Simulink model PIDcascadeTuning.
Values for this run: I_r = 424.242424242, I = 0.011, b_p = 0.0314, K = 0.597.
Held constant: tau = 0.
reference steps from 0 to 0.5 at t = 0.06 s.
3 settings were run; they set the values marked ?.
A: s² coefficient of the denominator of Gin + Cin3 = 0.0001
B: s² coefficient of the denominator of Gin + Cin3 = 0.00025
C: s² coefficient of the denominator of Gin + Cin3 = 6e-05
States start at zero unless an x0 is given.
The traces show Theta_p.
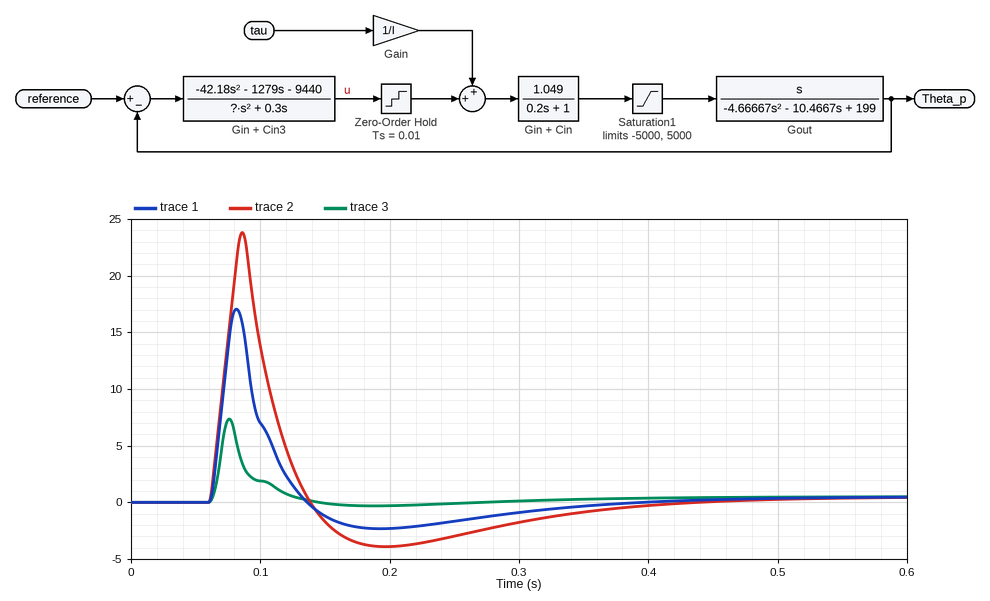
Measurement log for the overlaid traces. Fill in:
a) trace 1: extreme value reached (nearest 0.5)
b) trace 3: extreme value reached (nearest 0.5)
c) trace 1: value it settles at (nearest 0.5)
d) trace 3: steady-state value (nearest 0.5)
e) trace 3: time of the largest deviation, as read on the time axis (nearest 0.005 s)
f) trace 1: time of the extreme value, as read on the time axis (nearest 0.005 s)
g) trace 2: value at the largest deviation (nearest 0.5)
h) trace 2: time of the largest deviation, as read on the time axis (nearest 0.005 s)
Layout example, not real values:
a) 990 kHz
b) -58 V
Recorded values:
a) 17.0
b) 7.5
c) 0.5
d) 0.5
e) 0.075 s
f) 0.080 s
g) 24.0
h) 0.085 s
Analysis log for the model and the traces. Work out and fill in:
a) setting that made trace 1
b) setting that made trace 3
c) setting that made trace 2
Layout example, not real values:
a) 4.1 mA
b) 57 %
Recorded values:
a) A
b) B
c) C
